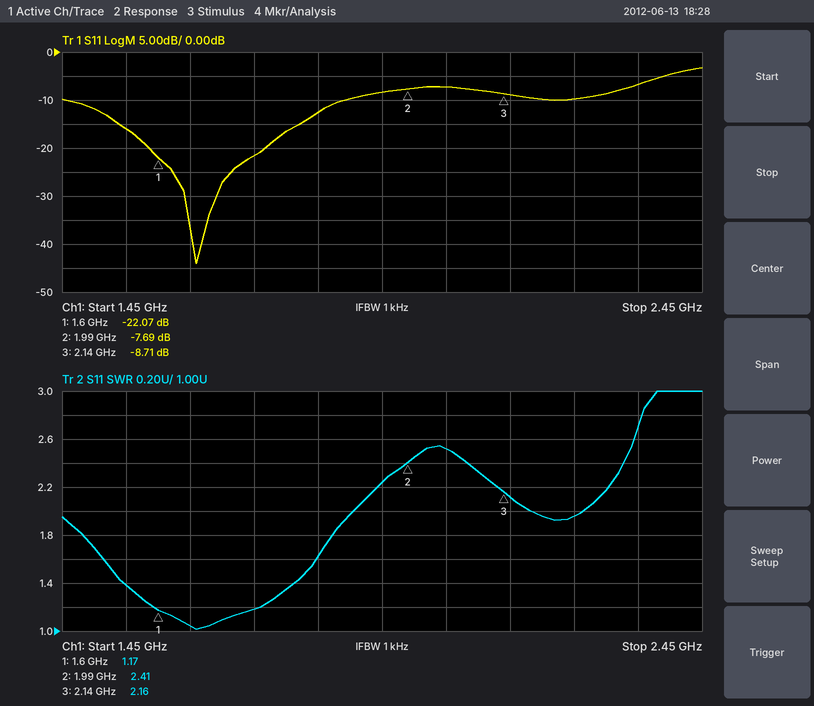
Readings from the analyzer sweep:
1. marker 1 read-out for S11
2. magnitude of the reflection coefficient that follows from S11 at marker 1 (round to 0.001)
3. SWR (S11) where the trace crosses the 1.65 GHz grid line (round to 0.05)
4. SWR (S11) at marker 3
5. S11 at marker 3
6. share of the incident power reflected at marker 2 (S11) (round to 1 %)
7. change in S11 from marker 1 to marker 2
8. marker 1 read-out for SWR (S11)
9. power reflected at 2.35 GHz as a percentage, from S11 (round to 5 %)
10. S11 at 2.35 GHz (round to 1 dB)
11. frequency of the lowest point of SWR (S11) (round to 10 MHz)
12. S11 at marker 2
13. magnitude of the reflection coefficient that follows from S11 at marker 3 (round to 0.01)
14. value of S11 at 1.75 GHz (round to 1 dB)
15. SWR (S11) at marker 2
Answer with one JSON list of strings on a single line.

["-22.07 dB", "0.079", "1.05", "2.16", "-8.71 dB", "17 %", "14.38 dB", "1.17", "20 %", "-7 dB", "1.66 GHz", "-7.69 dB", "0.37", "-22 dB", "2.41"]
